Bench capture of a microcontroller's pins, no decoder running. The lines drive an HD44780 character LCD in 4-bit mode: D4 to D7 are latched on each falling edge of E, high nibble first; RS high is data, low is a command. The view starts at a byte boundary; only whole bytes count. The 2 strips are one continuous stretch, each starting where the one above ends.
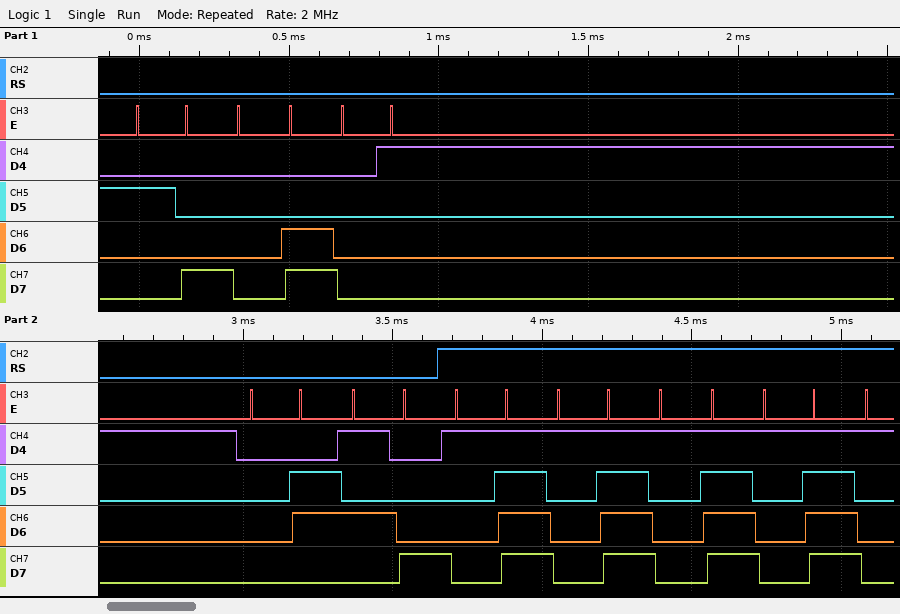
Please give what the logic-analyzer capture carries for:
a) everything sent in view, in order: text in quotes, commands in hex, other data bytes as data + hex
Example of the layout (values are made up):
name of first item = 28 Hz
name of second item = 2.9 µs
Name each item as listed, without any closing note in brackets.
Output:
everything sent in view, in order: text in quotes, commands in hex, other data bytes as data + hex = 0x28 0x0C 0x01 0x06 0x58 data 1F 1F 1F 1F
